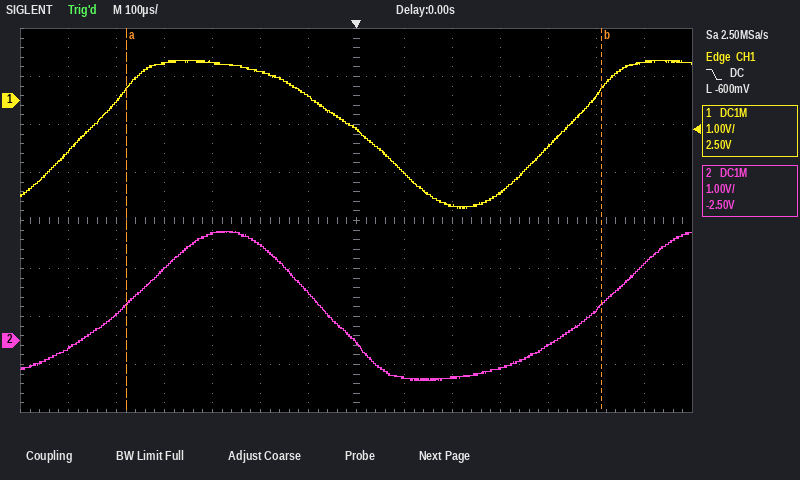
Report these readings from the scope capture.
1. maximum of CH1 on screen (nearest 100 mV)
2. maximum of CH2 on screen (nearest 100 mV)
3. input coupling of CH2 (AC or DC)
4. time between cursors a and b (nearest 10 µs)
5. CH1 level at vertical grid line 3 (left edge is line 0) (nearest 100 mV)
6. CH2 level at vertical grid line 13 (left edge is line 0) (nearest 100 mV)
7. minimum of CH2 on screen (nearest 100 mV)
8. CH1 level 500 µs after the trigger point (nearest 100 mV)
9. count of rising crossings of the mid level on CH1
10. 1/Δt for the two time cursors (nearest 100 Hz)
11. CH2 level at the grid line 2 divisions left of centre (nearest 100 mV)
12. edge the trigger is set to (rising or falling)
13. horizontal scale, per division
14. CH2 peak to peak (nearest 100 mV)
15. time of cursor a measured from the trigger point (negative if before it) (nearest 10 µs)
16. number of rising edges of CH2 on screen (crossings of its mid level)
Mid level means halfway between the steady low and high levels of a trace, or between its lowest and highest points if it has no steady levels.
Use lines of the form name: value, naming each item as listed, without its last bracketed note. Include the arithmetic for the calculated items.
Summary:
maximum of CH1 on screen: 800 mV
maximum of CH2 on screen: 2.3 V
input coupling of CH2: DC
time between cursors a and b: 990 µs
CH1 level at vertical grid line 3 (left edge is line 0): 800 mV
CH2 level at vertical grid line 13 (left edge is line 0): 1.6 V
minimum of CH2 on screen: -800 mV
CH1 level 500 µs after the trigger point: 100 mV
count of rising crossings of the mid level on CH1: 2
1/Δt for the two time cursors: 1 / 990 µs ≈ 1.0 kHz
CH2 level at the grid line 2 divisions left of centre: 2.0 V
edge the trigger is set to: falling
horizontal scale, per division: 100 µs
CH2 peak to peak: 2.3 V − (-800 mV) = 3.1 V
time of cursor a measured from the trigger point (negative if before it): -480 µs
number of rising edges of CH2 on screen: 2
